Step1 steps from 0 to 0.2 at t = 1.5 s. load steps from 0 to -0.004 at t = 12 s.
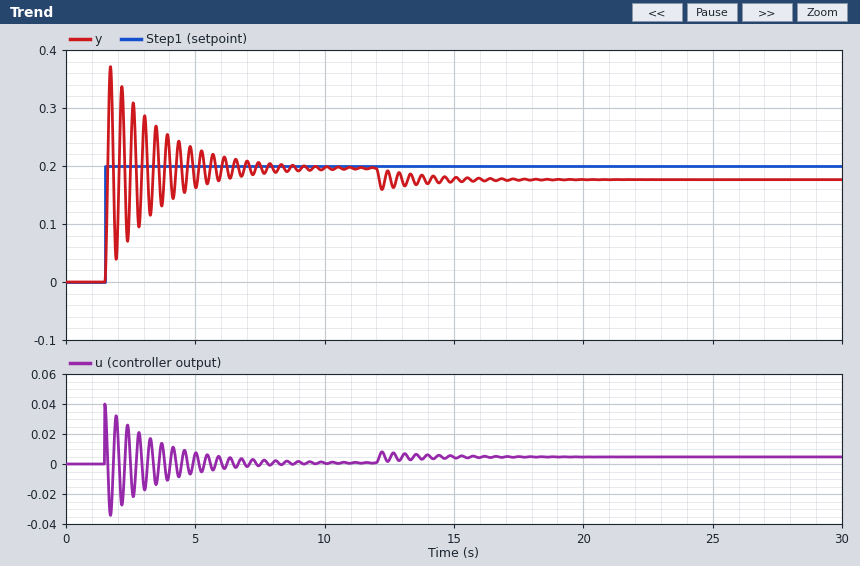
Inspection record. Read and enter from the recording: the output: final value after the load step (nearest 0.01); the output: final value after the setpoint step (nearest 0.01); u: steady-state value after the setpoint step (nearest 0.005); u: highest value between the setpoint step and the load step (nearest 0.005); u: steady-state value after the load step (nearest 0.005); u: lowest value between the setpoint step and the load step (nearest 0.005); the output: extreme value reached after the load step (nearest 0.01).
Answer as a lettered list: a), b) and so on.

a) 0.18
b) 0.20
c) 0.000
d) 0.040
e) 0.005
f) -0.035
g) 0.16
